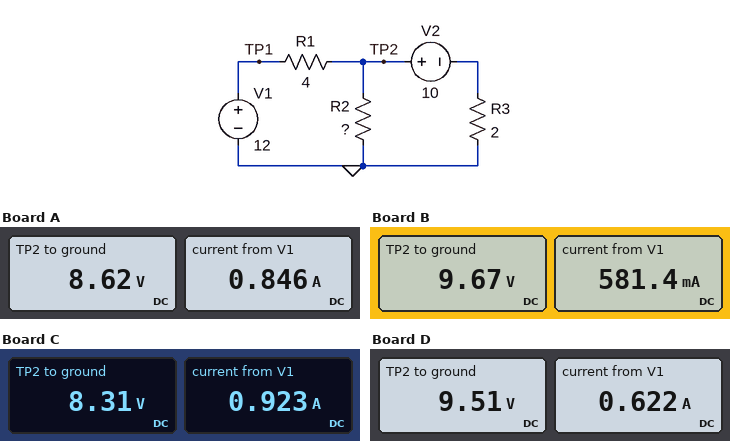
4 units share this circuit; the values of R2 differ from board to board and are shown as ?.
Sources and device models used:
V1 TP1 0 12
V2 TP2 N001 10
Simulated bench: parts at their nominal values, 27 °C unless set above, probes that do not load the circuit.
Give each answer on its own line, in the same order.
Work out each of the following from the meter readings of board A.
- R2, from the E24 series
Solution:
5.6 Ω
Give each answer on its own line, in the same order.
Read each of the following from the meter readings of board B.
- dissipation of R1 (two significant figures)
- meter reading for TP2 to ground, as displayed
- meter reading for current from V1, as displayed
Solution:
1.4 W
9.67 V
581.4 mA
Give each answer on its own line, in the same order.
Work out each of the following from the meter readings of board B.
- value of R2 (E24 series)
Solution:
13 Ω
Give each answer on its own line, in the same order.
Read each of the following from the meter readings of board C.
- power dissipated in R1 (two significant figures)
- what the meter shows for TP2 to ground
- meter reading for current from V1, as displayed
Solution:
3.4 W
8.31 V
0.923 A
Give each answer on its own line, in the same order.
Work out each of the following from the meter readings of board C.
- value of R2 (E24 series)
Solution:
4.7 Ω
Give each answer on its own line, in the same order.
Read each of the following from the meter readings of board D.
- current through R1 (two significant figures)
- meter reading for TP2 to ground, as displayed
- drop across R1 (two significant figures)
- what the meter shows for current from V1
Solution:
620 mA
9.51 V
2.5 V
0.622 A
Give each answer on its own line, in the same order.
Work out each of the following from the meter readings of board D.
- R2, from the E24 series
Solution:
11 Ω
